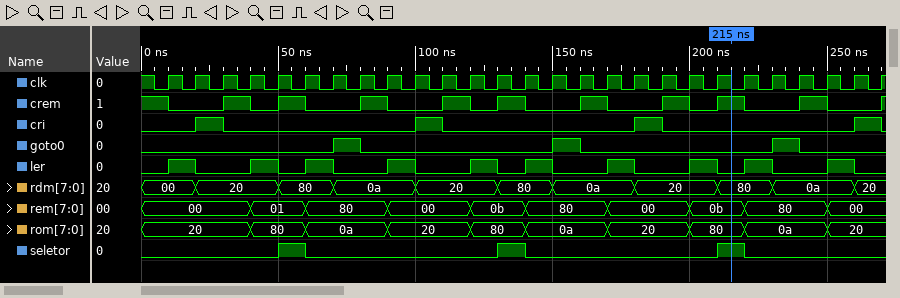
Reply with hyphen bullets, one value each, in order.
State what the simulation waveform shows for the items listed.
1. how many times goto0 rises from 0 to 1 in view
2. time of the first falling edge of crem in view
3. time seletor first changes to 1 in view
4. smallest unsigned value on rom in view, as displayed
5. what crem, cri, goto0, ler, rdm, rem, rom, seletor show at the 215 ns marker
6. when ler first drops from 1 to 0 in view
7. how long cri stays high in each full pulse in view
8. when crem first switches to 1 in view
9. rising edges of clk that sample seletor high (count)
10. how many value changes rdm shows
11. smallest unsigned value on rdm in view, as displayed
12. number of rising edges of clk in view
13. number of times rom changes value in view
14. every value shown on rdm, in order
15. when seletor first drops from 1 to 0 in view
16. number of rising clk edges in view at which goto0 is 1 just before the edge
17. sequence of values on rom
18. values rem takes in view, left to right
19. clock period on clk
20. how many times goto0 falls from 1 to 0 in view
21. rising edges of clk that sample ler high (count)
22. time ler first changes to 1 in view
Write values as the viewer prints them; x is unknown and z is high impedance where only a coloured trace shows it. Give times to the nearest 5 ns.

- 3
- 10 ns
- 50 ns
- 0a
- crem=1, cri=0, goto0=0, ler=0, rdm=80, rem=0b, rom=80, seletor=1
- 20 ns
- 10 ns, 10 ns, 10 ns, 10 ns
- 30 ns
- 3
- 10
- 00
- 27
- 9
- 00, 20, 80, 0a, 20, 80, 0a, 20, 80, 0a, 20
- 60 ns
- 3
- 20, 80, 0a, 20, 80, 0a, 20, 80, 0a, 20
- 00, 01, 80, 00, 0b, 80, 00, 0b, 80, 00
- 10 ns
- 3
- 10
- 10 ns
